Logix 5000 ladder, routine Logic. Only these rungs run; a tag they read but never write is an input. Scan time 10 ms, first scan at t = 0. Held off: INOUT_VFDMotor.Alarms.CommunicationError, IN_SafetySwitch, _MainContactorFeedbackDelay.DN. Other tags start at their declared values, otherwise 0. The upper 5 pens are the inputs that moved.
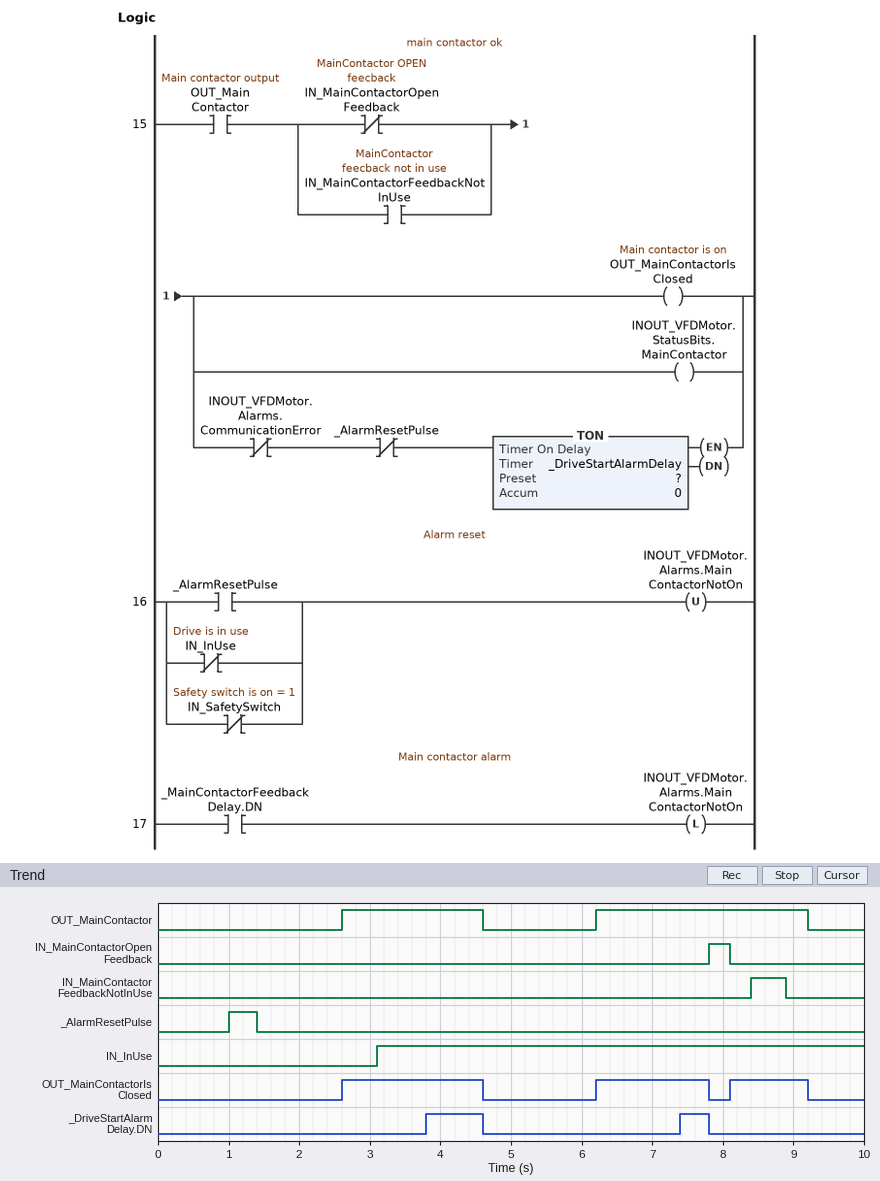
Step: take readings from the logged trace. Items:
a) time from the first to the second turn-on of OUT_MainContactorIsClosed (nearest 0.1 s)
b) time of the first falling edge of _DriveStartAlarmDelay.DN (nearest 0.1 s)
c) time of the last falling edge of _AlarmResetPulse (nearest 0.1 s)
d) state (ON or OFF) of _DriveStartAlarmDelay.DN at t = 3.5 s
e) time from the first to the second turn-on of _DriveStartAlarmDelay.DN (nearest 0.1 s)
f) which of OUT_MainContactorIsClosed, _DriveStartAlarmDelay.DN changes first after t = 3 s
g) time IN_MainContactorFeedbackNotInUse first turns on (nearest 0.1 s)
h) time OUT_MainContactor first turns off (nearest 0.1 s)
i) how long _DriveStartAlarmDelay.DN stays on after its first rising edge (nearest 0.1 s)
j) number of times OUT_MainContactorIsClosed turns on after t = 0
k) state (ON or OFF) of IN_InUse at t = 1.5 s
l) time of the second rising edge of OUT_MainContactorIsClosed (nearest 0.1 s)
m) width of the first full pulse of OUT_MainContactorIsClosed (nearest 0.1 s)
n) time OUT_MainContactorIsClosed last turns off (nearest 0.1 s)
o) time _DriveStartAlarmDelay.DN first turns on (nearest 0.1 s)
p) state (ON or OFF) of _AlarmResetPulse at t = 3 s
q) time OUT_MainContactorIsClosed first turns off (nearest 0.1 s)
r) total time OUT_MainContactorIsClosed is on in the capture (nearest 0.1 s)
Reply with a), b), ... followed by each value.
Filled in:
a) 3.6 s
b) 4.6 s
c) 1.4 s
d) OFF
e) 3.6 s
f) _DriveStartAlarmDelay.DN
g) 8.4 s
h) 4.6 s
i) 0.8 s
j) 3
k) OFF
l) 6.2 s
m) 2.0 s
n) 9.2 s
o) 3.8 s
p) OFF
q) 4.6 s
r) 4.7 s
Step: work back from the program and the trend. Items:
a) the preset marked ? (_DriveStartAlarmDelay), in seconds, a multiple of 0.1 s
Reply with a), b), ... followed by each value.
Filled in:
a) 1.2 s
